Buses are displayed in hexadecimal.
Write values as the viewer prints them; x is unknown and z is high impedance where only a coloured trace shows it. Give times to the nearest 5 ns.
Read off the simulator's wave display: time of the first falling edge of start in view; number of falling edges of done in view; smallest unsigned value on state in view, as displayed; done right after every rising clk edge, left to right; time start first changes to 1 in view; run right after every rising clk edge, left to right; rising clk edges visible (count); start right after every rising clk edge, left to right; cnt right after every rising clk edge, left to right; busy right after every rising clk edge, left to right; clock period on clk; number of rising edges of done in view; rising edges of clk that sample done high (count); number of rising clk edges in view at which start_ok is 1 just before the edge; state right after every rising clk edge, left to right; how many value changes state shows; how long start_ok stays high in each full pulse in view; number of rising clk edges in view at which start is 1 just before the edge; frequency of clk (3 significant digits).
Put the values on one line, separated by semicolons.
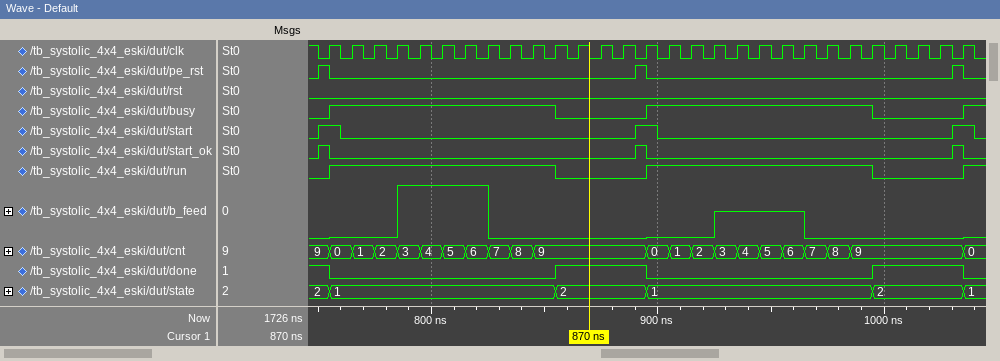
760 ns; 3; 1; 0 0 0 0 0 0 0 0 0 0 1 1 1 1 0 0 0 0 0 0 0 0 0 0 1 1 1 1 0; 750 ns; 1 1 1 1 1 1 1 1 1 1 0 0 0 0 1 1 1 1 1 1 1 1 1 1 0 0 0 0 1; 29; 1 0 0 0 0 0 0 0 0 0 0 0 0 0 1 0 0 0 0 0 0 0 0 0 0 0 0 0 1; 0, 1, 2, 3, 4, 5, 6, 7, 8, 9, 9, 9, 9, 9, 0, 1, 2, 3, 4, 5, 6, 7, 8, 9, 9, 9, 9, 9, 0; 1 1 1 1 1 1 1 1 1 1 0 0 0 0 1 1 1 1 1 1 1 1 1 1 0 0 0 0 1; 10 ns; 2; 9; 3; 1, 1, 1, 1, 1, 1, 1, 1, 1, 1, 2, 2, 2, 2, 1, 1, 1, 1, 1, 1, 1, 1, 1, 1, 2, 2, 2, 2, 1; 5; 5 ns, 5 ns, 5 ns; 3; 100 MHz
